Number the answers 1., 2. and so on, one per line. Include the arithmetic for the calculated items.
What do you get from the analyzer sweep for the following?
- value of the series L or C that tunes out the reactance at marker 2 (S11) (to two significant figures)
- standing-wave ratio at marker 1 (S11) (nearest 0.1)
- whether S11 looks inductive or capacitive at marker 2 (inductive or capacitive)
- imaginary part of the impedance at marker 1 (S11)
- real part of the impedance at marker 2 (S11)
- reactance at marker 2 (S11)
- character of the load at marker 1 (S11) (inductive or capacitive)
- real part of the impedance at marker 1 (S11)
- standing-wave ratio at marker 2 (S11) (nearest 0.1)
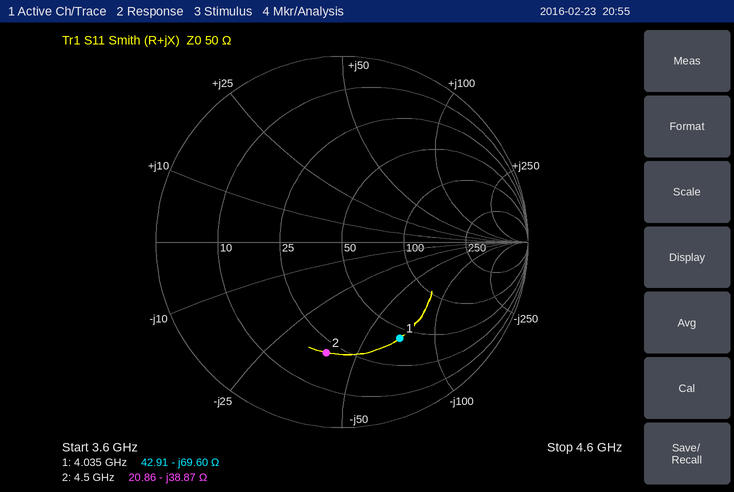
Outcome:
1. L = 38.87 Ω/(2π × 4.5 GHz) ≈ 1.4 nH
2. 4.0
3. capacitive
4. -69.60 Ω
5. 20.86 Ω
6. -38.87 Ω
7. capacitive
8. 42.91 Ω
9. 4.0
